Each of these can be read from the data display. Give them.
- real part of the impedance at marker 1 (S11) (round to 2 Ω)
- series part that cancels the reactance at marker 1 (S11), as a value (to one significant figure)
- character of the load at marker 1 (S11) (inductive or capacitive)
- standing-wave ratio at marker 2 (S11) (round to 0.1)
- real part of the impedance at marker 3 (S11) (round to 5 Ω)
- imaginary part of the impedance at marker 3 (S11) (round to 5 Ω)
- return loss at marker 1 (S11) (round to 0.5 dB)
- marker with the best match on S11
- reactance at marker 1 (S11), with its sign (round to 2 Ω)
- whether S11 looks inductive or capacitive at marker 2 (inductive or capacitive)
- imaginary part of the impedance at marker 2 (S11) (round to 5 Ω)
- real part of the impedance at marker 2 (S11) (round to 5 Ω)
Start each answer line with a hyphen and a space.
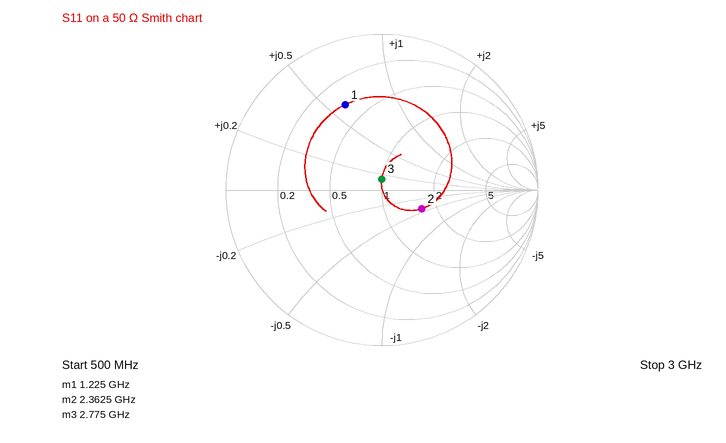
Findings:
- 18 Ω
- 4 pF
- inductive
- 1.8
- 50 Ω
- +5 Ω
- 4.5 dB
- marker 3
- +30 Ω
- capacitive
- -20 Ω
- 80 Ω
